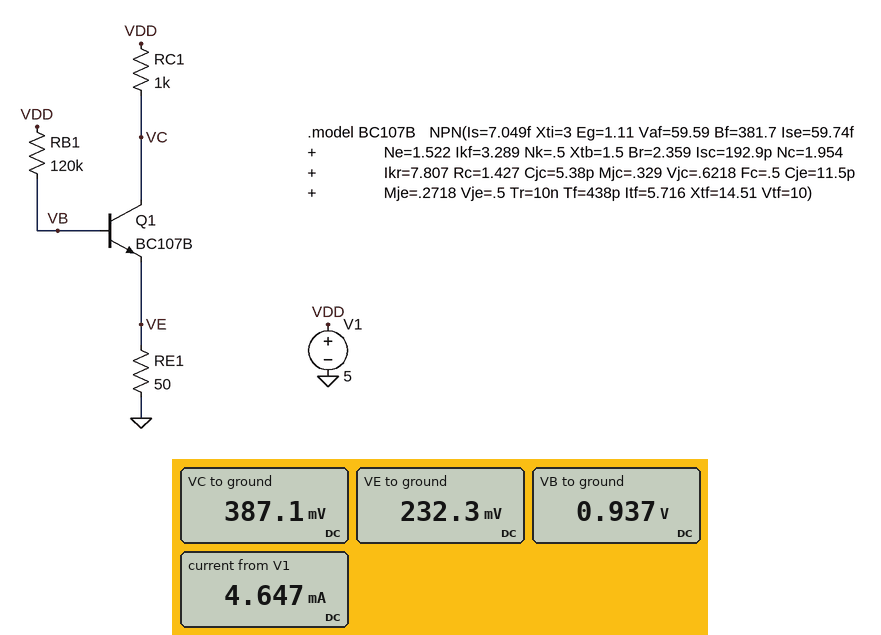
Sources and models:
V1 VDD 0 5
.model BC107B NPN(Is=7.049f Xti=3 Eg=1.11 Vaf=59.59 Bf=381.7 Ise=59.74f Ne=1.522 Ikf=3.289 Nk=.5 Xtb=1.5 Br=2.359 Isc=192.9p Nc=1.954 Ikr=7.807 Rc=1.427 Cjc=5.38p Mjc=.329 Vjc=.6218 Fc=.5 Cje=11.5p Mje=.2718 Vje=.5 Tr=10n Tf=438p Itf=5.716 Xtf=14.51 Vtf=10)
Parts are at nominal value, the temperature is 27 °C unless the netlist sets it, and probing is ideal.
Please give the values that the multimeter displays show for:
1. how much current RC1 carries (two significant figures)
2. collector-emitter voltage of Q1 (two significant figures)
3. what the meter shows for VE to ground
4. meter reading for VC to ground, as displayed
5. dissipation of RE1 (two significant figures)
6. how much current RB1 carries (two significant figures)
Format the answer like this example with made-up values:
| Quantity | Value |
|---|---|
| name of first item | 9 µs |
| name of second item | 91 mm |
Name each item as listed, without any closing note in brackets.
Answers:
| Quantity | Value |
|---|---|
| how much current RC1 carries | 4.6 mA |
| collector-emitter voltage of Q1 | 150 mV |
| what the meter shows for VE to ground | 232.3 mV |
| meter reading for VC to ground, as displayed | 387.1 mV |
| dissipation of RE1 | 1.1 mW |
| how much current RB1 carries | 34 µA |
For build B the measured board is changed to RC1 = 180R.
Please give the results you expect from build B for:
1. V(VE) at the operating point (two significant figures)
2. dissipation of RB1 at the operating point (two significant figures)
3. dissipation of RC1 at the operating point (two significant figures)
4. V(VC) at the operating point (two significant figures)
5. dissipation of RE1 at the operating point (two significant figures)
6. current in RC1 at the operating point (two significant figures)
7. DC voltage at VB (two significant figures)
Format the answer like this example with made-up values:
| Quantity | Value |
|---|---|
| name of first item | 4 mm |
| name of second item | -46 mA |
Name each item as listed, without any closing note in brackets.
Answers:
| Quantity | Value |
|---|---|
| V(VE) at the operating point | 510 mV |
| dissipation of RB1 at the operating point | 120 µW |
| dissipation of RC1 at the operating point | 18 mW |
| V(VC) at the operating point | 3.2 V |
| dissipation of RE1 at the operating point | 5.1 mW |
| current in RC1 at the operating point | 10 mA |
| DC voltage at VB | 1.2 V |
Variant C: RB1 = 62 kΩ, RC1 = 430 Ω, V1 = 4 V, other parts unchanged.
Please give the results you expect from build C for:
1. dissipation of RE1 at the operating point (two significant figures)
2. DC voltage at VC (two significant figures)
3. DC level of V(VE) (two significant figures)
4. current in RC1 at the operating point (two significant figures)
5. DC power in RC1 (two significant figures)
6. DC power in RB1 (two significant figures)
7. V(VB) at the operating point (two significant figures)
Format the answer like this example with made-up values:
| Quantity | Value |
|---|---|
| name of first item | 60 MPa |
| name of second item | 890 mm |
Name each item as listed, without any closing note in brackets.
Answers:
| Quantity | Value |
|---|---|
| dissipation of RE1 at the operating point | 3.2 mW |
| DC voltage at VC | 570 mV |
| DC level of V(VE) | 400 mV |
| current in RC1 at the operating point | 8.0 mA |
| DC power in RC1 | 27 mW |
| DC power in RB1 | 130 µW |
| V(VB) at the operating point | 1.1 V |
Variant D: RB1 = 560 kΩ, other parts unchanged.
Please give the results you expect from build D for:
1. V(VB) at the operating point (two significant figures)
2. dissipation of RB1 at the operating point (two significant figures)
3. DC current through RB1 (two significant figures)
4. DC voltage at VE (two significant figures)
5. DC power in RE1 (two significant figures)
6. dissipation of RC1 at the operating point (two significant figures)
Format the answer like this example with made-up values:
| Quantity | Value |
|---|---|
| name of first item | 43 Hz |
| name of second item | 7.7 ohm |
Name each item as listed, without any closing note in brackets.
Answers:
| Quantity | Value |
|---|---|
| V(VB) at the operating point | 790 mV |
| dissipation of RB1 at the operating point | 32 µW |
| DC current through RB1 | 7.5 µA |
| DC voltage at VE | 110 mV |
| DC power in RE1 | 230 µW |
| dissipation of RC1 at the operating point | 4.6 mW |
